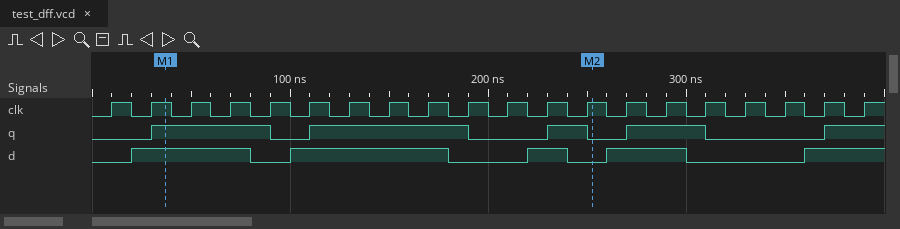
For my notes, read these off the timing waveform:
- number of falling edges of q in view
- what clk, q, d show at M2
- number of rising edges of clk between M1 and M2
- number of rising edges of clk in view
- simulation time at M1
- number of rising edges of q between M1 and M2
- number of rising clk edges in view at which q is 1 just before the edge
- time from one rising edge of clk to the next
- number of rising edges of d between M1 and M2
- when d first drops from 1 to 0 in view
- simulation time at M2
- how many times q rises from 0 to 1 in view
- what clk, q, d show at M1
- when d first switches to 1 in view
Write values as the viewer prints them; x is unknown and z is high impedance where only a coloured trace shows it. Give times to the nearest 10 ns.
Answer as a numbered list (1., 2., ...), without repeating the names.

1. 4
2. clk=1, q=0, d=0
3. 11
4. 20
5. 40 ns
6. 2
7. 11
8. 20 ns
9. 2
10. 80 ns
11. 250 ns
12. 5
13. clk=1, q=1, d=1
14. 20 ns
